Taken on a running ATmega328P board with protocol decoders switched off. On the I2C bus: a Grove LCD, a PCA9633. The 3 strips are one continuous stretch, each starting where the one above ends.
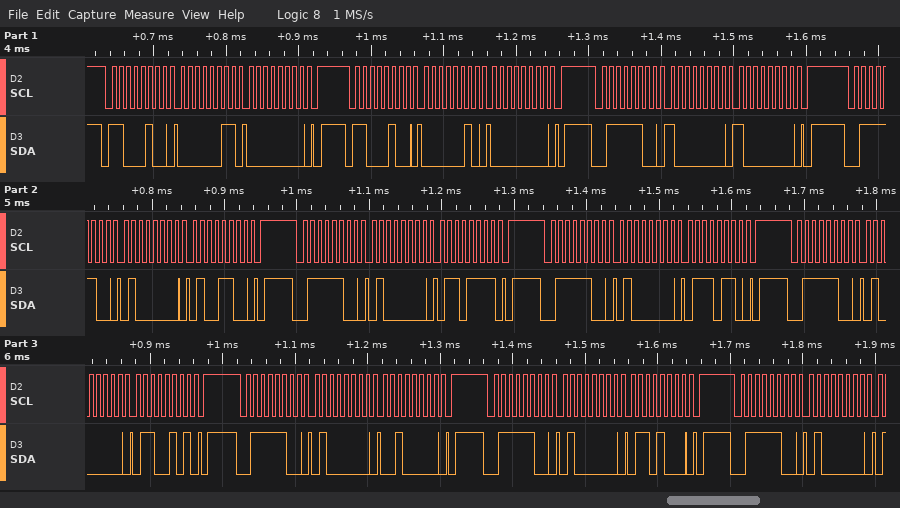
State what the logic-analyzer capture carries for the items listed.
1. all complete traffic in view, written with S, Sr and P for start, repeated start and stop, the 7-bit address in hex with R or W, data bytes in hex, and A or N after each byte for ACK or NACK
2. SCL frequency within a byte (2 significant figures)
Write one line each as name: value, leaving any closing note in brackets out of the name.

all complete traffic in view, written with S, Sr and P for start, repeated start and stop, the 7-bit address in hex with R or W, data bytes in hex, and A or N after each byte for ACK or NACK: S 62W A 03 A 00 A P S 62W A 02 A 00 A P S 3EW A 80 A 80 A P S 3EW A 40 A 4C A P S 3EW A 40 A 6F A P S 3EW A 40 A 76 A P S 3EW A 40 A 65 A P S 3EW A 40 A 20 A P S 3EW A 40 A 68 A P S 3EW A 40 A
SCL frequency within a byte: 100 kHz
